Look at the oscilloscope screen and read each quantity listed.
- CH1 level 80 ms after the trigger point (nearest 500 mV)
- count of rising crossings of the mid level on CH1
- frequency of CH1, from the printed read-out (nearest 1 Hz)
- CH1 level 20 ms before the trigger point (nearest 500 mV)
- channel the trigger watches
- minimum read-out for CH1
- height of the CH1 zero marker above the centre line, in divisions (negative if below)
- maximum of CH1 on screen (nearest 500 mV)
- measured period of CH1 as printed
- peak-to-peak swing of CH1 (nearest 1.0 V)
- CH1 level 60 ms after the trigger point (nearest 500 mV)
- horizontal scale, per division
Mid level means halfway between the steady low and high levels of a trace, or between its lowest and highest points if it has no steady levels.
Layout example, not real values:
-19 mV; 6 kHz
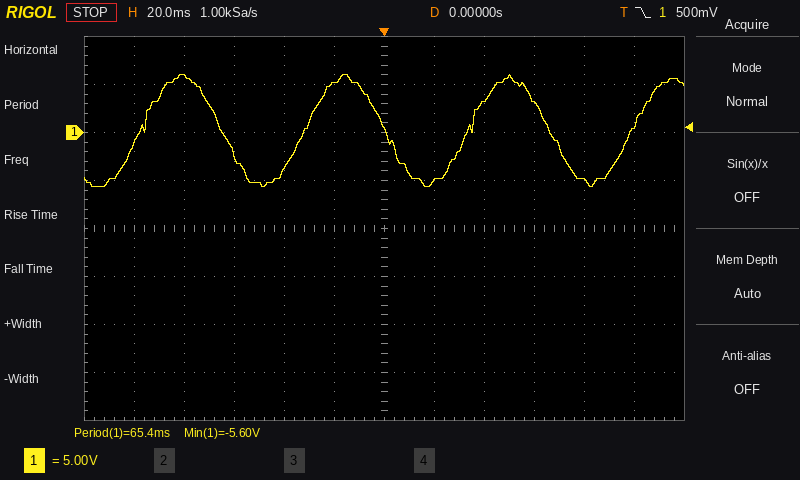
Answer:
-5.0 V; 4; 15 Hz; 5.0 V; CH1; -5.60 V; +2.0 div; 6.0 V; 65.4 ms; 12.0 V; 3.0 V; 20 ms
